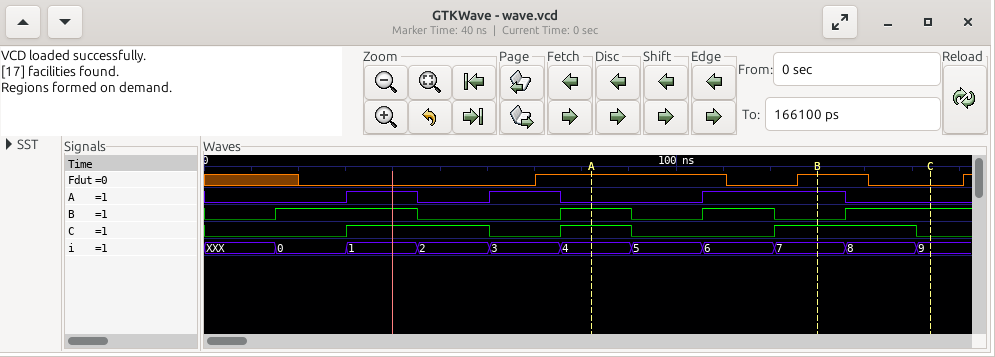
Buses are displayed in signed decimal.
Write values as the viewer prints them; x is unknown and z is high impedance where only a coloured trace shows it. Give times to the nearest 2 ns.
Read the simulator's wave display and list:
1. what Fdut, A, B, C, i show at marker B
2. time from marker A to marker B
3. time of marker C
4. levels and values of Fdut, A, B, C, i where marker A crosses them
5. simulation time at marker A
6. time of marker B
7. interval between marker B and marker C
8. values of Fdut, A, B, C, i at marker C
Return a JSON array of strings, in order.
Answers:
["Fdut=1, A=1, B=0, C=1, i=7", "48 ns", "154 ns", "Fdut=1, A=0, B=1, C=1, i=4", "82 ns", "130 ns", "24 ns", "Fdut=0, A=0, B=1, C=0, i=9"]
